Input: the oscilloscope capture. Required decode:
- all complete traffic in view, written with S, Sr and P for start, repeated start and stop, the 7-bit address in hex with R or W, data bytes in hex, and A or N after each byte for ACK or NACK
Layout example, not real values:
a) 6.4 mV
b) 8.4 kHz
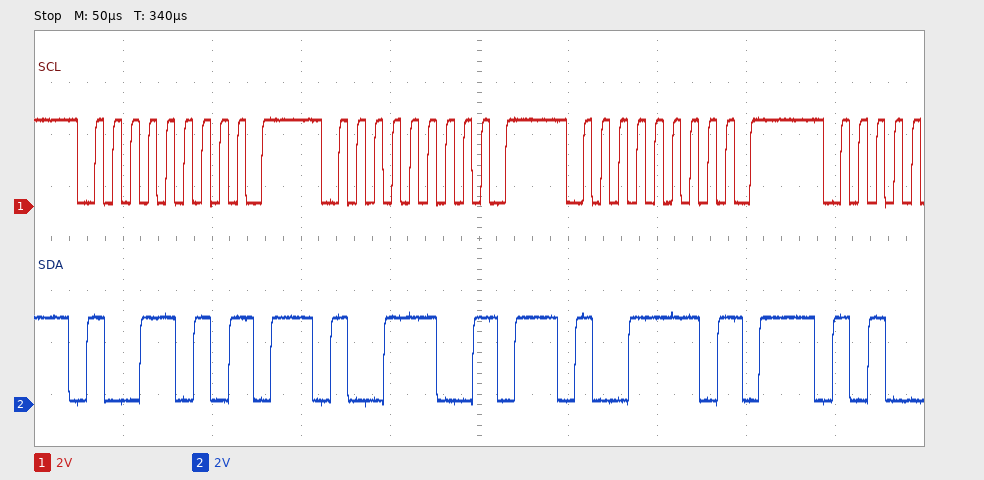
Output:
a) S 4DW N P S 4EW N P S 4FW N P
